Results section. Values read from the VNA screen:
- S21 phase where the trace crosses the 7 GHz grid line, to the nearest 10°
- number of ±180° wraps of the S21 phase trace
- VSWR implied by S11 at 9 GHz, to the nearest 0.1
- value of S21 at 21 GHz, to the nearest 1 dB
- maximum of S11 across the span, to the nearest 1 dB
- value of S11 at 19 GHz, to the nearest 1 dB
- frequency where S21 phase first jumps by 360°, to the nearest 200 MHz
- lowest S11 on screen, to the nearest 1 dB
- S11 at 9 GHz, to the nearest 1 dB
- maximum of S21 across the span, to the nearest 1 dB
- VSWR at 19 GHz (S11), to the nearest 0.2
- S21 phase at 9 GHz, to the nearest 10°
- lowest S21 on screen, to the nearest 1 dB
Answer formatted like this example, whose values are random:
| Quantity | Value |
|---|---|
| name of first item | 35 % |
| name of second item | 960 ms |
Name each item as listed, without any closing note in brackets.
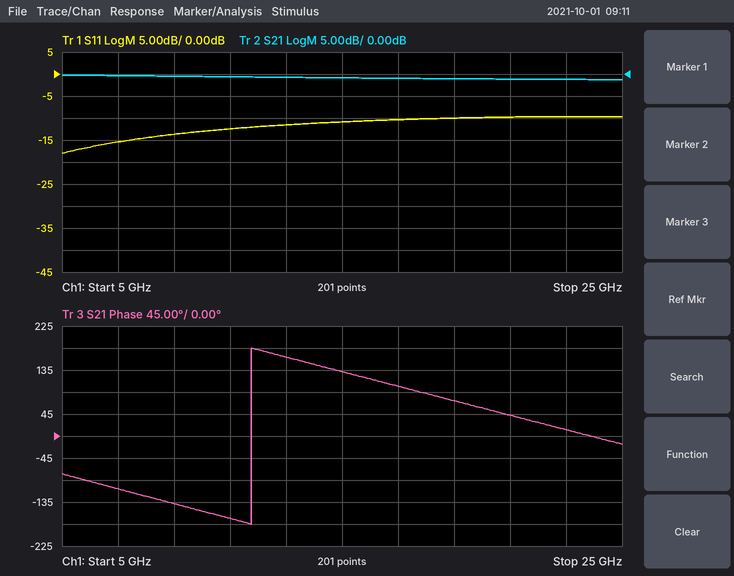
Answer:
| Quantity | Value |
|---|---|
| S21 phase where the trace crosses the 7 GHz grid line, to the nearest 10° | -110° |
| number of ±180° wraps of the S21 phase trace | 1 |
| VSWR implied by S11 at 9 GHz, to the nearest 0.1 | 1.5 |
| value of S21 at 21 GHz, to the nearest 1 dB | -1 dB |
| maximum of S11 across the span, to the nearest 1 dB | -10 dB |
| value of S11 at 19 GHz, to the nearest 1 dB | -10 dB |
| frequency where S21 phase first jumps by 360°, to the nearest 200 MHz | 11.8 GHz |
| lowest S11 on screen, to the nearest 1 dB | -18 dB |
| S11 at 9 GHz, to the nearest 1 dB | -14 dB |
| maximum of S21 across the span, to the nearest 1 dB | 0 dB |
| VSWR at 19 GHz (S11), to the nearest 0.2 | 2.0 |
| S21 phase at 9 GHz, to the nearest 10° | -140° |
| lowest S21 on screen, to the nearest 1 dB | -1 dB |
